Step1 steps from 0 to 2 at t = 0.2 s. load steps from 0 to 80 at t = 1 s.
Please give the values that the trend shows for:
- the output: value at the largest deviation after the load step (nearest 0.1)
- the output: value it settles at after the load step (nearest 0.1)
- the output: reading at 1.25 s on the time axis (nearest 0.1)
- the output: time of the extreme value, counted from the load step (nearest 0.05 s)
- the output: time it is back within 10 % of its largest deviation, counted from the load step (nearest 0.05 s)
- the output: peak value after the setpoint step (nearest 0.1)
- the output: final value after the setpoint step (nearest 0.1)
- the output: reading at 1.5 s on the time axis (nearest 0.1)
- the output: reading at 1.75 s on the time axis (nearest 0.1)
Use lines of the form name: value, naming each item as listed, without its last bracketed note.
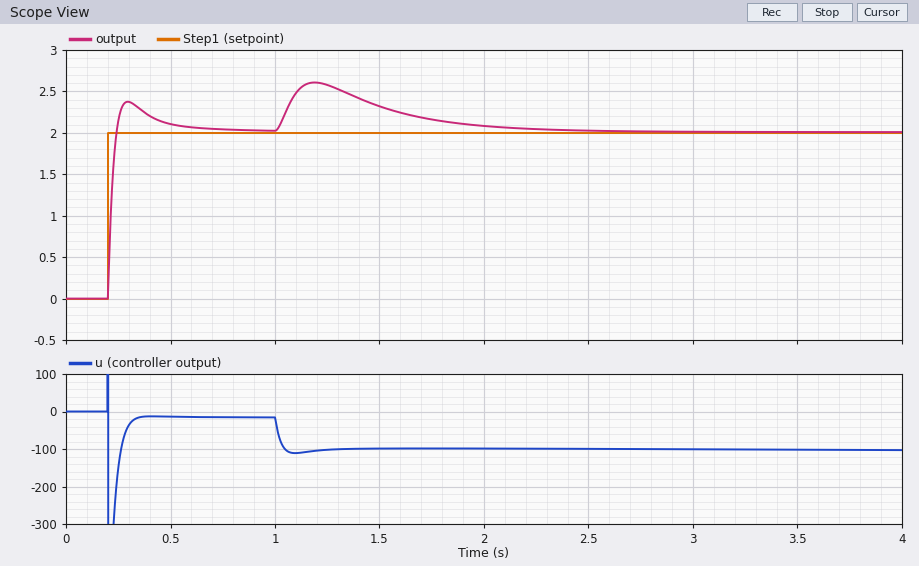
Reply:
the output: value at the largest deviation after the load step: 2.6
the output: value it settles at after the load step: 2.0
the output: reading at 1.25 s on the time axis: 2.6
the output: time of the extreme value, counted from the load step: 0.20 s
the output: time it is back within 10 % of its largest deviation, counted from the load step: 1.10 s
the output: peak value after the setpoint step: 2.4
the output: final value after the setpoint step: 2.0
the output: reading at 1.5 s on the time axis: 2.3
the output: reading at 1.75 s on the time axis: 2.2
